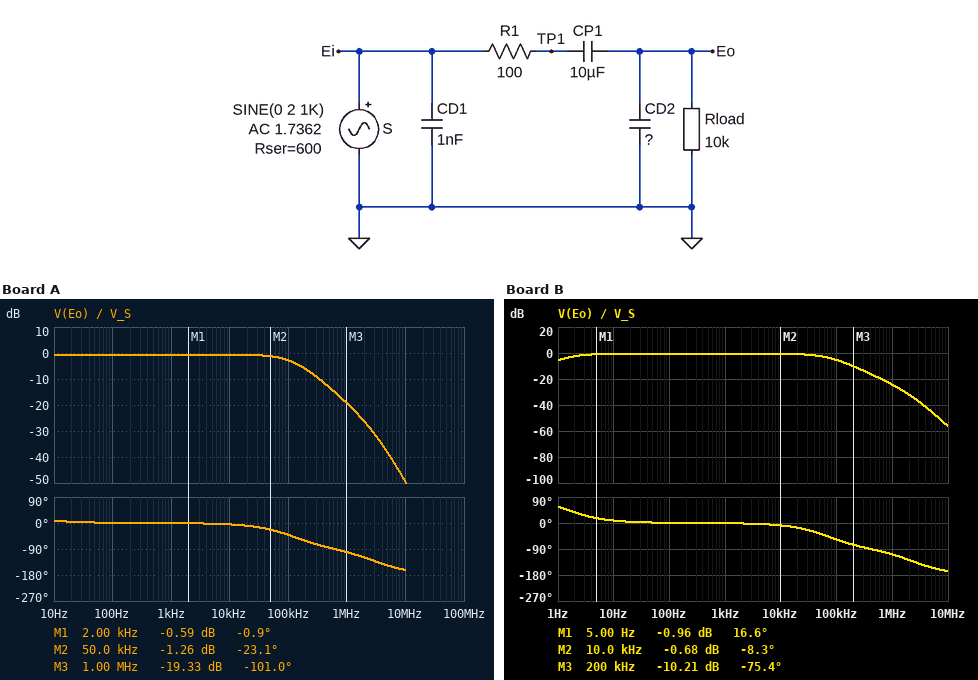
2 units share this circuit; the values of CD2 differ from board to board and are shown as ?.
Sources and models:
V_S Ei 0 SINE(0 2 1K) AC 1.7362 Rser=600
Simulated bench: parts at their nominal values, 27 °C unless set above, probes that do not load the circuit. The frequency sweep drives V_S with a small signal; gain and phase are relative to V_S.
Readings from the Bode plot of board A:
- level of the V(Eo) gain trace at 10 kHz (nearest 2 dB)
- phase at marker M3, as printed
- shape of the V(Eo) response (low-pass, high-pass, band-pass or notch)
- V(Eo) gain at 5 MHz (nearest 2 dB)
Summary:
0 dB
-101.0 deg
low-pass
-38 dB
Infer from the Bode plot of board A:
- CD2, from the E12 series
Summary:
1.2 nF
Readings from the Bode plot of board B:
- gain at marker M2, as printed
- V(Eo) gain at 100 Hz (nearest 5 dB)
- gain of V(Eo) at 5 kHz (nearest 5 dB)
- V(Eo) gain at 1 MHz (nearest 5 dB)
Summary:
-0.68 dB
0 dB
0 dB
-25 dB
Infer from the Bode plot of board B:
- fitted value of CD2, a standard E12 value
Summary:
2.7 nF
